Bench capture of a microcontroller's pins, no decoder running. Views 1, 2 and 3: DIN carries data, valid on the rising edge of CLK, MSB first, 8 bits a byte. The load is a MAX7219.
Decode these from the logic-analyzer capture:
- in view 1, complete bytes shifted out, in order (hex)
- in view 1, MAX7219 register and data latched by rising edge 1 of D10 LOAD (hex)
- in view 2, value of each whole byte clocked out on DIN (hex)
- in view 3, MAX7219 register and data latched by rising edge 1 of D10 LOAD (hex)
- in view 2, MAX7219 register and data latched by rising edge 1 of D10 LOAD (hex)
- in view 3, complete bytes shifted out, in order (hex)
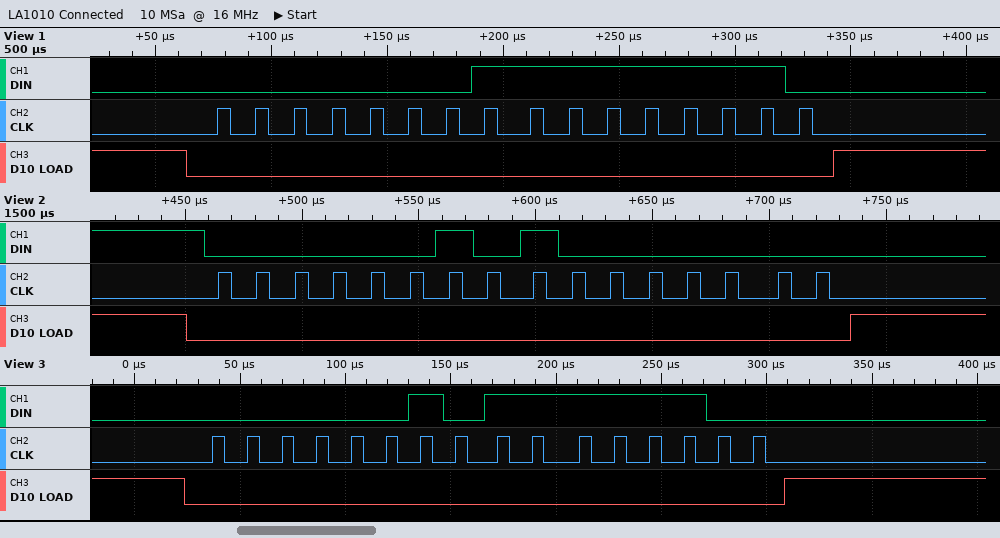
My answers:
01 FE
register 0x1, data 0xFE
0x02 0x80
register 0x2, data 0xFC
register 0x2, data 0x80
02 FC
